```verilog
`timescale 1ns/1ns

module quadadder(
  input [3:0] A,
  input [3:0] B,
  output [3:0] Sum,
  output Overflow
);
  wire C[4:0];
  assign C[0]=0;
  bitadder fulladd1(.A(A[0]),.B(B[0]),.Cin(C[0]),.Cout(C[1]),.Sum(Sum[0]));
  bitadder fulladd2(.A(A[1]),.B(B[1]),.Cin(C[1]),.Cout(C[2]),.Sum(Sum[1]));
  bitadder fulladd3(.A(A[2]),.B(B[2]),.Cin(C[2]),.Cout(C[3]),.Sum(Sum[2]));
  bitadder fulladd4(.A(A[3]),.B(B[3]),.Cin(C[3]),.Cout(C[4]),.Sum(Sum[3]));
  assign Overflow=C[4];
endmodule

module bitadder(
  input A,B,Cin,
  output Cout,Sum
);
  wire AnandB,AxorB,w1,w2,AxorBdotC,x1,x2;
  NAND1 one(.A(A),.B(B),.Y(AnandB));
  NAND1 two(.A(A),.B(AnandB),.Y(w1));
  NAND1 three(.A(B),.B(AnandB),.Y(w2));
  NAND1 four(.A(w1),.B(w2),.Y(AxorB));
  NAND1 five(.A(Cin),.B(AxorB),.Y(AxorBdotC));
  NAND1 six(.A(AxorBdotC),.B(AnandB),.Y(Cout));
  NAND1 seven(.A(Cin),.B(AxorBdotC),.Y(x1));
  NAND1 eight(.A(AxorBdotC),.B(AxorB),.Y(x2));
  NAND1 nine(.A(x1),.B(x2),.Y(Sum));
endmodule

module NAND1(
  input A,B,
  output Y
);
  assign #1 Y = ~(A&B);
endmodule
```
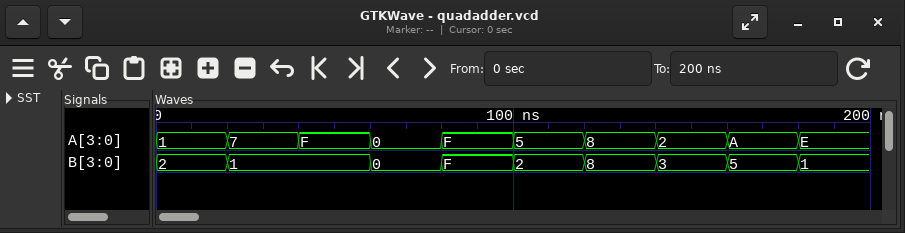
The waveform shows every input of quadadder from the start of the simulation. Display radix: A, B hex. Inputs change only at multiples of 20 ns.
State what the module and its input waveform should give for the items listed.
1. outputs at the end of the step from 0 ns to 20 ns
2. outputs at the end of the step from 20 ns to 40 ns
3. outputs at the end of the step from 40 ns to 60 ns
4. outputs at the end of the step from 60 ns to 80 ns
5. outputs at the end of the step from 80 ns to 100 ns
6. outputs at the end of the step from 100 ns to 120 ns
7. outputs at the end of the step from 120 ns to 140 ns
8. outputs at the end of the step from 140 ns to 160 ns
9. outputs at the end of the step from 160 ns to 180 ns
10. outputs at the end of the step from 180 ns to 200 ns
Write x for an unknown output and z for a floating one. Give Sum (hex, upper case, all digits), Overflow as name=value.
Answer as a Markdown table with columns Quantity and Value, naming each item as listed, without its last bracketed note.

| Quantity | Value |
|---|---|
| outputs at the end of the step from 0 ns to 20 ns | Sum=3, Overflow=0 |
| outputs at the end of the step from 20 ns to 40 ns | Sum=8, Overflow=0 |
| outputs at the end of the step from 40 ns to 60 ns | Sum=0, Overflow=1 |
| outputs at the end of the step from 60 ns to 80 ns | Sum=0, Overflow=0 |
| outputs at the end of the step from 80 ns to 100 ns | Sum=E, Overflow=1 |
| outputs at the end of the step from 100 ns to 120 ns | Sum=7, Overflow=0 |
| outputs at the end of the step from 120 ns to 140 ns | Sum=0, Overflow=1 |
| outputs at the end of the step from 140 ns to 160 ns | Sum=5, Overflow=0 |
| outputs at the end of the step from 160 ns to 180 ns | Sum=F, Overflow=0 |
| outputs at the end of the step from 180 ns to 200 ns | Sum=F, Overflow=0 |
